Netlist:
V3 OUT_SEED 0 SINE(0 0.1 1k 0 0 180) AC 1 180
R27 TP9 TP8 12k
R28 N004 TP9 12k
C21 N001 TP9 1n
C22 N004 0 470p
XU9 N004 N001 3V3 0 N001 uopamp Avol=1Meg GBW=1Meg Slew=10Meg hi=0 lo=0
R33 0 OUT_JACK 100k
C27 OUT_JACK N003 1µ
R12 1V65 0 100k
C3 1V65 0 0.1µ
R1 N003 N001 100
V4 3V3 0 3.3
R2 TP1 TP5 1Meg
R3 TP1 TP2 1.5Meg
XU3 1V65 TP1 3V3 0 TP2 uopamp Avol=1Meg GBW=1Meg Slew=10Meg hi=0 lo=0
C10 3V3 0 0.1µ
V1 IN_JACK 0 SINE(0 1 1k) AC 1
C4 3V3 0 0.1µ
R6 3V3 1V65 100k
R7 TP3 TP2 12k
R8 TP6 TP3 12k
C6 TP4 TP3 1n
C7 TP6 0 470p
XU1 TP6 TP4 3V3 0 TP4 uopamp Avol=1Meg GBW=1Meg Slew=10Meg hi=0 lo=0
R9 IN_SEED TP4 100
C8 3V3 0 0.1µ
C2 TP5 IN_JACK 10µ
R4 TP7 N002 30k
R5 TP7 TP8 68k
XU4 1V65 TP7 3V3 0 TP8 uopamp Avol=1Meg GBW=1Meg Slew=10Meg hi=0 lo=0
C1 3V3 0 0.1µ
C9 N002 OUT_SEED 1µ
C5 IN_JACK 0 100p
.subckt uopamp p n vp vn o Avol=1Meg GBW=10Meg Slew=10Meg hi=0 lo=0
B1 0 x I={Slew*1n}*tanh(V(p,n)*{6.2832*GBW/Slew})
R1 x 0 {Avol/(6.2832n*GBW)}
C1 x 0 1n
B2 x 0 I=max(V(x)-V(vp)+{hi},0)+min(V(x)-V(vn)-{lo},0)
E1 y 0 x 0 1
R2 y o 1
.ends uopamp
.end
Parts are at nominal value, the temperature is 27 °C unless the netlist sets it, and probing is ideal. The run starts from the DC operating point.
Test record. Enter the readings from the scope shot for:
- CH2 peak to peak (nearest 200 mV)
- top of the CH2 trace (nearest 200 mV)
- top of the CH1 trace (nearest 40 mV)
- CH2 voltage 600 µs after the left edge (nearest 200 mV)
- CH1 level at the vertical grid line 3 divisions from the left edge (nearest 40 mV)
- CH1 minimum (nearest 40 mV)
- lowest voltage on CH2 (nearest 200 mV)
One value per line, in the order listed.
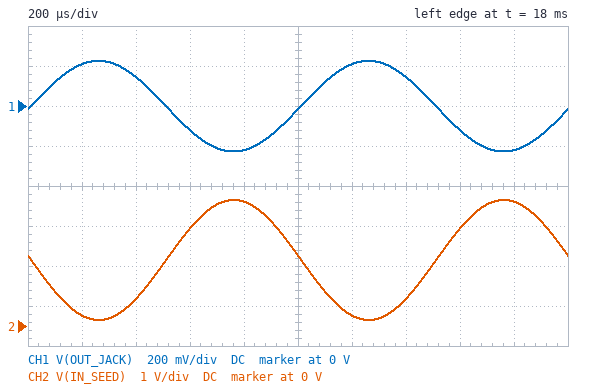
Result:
3.0 V
3.2 V
240 mV
2.4 V
-120 mV
-240 mV
200 mV
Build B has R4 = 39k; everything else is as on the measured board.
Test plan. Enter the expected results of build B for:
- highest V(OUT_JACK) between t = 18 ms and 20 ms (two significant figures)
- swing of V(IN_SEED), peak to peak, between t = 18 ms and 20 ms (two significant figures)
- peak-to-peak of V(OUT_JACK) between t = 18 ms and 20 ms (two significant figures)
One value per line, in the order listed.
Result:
170 mV
3.0 V
350 mV
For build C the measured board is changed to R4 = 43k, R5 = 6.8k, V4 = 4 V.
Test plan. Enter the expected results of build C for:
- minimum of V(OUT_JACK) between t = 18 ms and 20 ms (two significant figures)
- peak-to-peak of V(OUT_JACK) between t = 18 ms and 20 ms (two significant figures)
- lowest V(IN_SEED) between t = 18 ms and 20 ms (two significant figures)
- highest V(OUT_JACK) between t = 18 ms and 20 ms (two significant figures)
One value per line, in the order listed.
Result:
-16 mV
32 mV
500 mV
16 mV
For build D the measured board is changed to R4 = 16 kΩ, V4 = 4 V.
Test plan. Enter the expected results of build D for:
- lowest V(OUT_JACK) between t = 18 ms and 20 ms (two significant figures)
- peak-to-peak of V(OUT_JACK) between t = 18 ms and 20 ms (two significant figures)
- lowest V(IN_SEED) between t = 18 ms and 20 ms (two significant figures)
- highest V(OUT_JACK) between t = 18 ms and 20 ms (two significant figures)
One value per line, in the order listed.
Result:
-430 mV
850 mV
500 mV
420 mV
